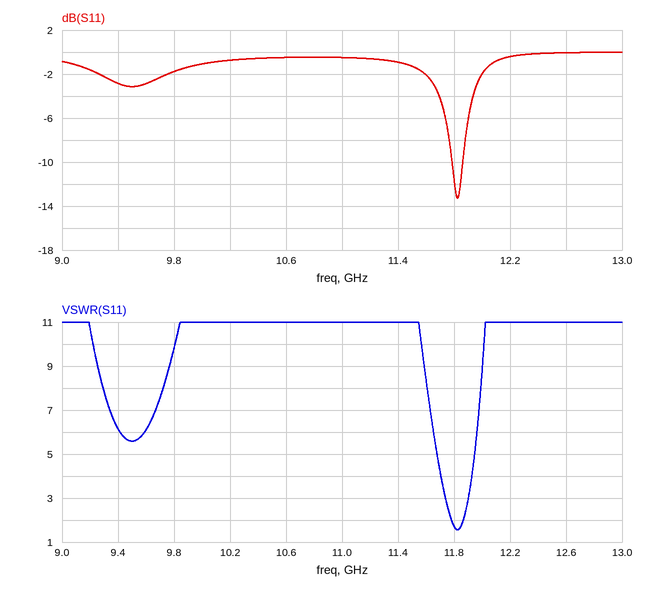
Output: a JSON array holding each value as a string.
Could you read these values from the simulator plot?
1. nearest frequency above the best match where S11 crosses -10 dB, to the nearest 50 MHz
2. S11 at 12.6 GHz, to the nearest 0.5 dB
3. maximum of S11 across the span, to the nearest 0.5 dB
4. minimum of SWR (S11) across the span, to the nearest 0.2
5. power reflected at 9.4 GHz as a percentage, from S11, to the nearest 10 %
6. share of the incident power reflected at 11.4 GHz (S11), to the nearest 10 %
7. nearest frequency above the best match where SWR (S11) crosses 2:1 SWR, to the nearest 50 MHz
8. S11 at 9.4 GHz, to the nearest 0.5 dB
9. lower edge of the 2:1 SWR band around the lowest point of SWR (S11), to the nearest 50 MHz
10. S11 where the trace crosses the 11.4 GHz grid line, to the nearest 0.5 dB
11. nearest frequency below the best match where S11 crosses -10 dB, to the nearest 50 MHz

["11.85 GHz", "0.0 dB", "0.0 dB", "1.6", "50 %", "80 %", "11.85 GHz", "-3.0 dB", "11.80 GHz", "-1.0 dB", "11.80 GHz"]
